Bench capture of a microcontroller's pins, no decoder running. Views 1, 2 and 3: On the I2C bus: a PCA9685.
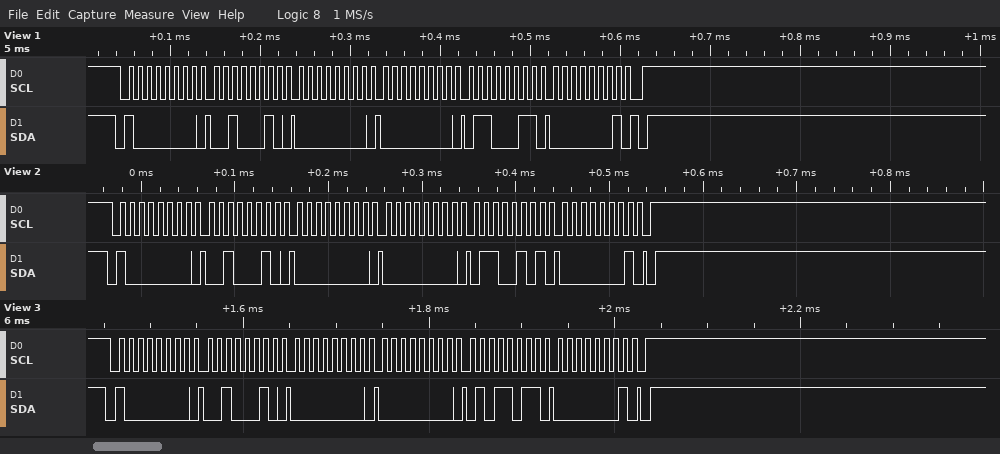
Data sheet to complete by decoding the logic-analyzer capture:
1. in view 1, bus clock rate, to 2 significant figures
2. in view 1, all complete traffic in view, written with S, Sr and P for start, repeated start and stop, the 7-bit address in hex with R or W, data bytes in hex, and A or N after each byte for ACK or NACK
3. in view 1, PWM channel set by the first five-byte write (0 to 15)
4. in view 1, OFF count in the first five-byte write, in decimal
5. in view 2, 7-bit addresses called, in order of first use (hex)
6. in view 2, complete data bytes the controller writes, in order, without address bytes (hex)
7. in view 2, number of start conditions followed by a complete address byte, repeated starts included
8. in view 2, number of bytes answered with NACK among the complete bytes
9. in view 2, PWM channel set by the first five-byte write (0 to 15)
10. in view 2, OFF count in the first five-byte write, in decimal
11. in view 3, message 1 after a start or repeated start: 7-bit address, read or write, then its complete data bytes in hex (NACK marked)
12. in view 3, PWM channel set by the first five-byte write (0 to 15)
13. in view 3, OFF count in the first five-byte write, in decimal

100 kHz
S 40W A 22 A 00 A 00 A 63 A 01 A P
7
355
0x40
22 00 00 65 01
1
0
7
357
0x40 write: 22 00 00 5B 01
7
347
